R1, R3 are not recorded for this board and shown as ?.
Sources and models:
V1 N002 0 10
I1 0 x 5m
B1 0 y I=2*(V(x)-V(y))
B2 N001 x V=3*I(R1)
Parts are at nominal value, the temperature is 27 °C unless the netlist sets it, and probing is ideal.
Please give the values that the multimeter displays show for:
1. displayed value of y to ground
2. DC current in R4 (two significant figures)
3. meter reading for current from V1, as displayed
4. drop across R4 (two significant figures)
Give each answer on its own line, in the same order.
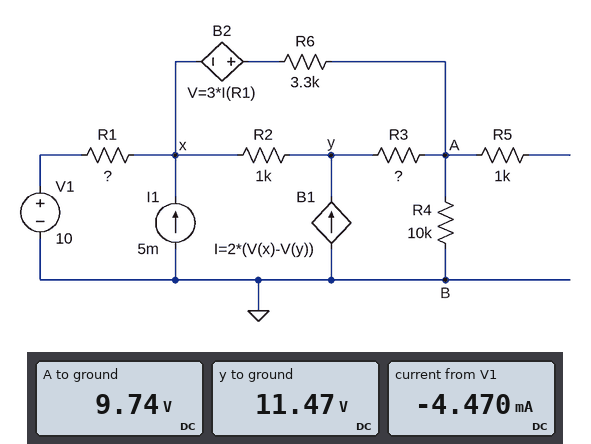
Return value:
11.47 V
970 µA
-4.470 mA
9.7 V
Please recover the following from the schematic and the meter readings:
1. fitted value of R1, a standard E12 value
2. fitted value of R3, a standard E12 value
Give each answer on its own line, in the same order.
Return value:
330 Ω
3.9 kΩ
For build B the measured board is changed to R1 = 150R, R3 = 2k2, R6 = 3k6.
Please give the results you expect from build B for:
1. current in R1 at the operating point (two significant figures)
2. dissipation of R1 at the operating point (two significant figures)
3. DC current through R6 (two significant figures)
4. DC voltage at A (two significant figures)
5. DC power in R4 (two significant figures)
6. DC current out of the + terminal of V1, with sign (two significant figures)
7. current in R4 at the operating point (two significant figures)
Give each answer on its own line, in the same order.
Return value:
4.6 mA
3.2 mW
360 µA
9.4 V
8.9 mW
-4.6 mA
940 µA
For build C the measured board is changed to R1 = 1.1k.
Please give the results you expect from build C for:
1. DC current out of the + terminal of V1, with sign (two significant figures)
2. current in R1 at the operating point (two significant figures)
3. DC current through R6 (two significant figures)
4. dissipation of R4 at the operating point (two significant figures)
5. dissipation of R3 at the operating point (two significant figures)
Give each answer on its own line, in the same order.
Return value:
-4.3 mA
4.3 mA
680 µA
16 mW
1.3 mW
